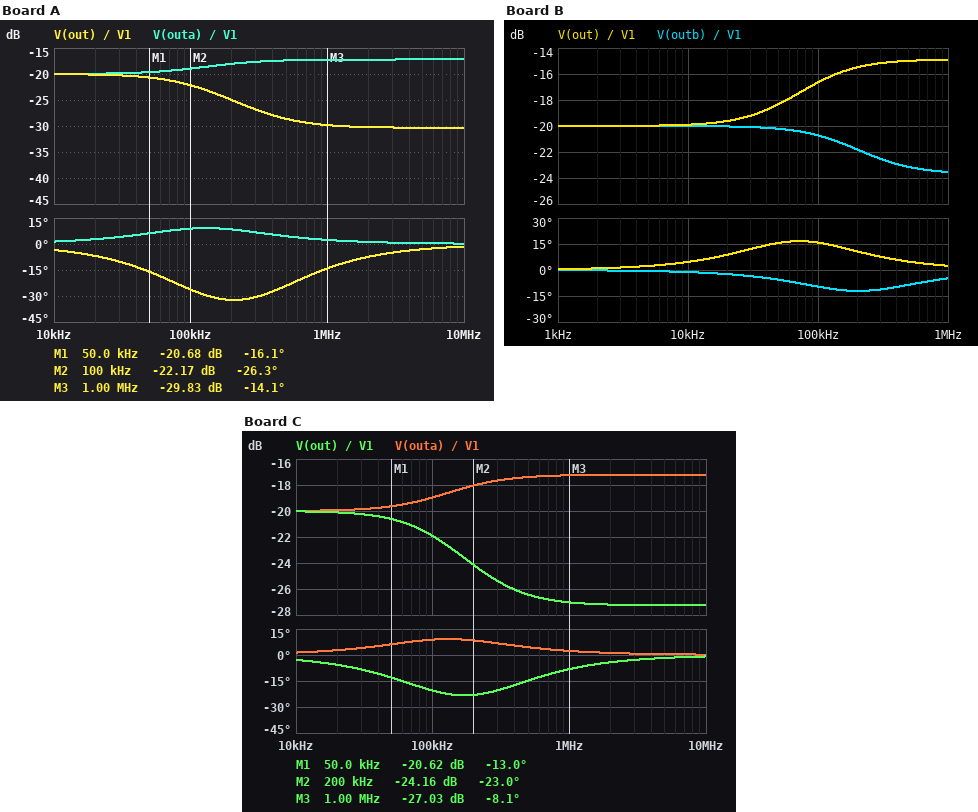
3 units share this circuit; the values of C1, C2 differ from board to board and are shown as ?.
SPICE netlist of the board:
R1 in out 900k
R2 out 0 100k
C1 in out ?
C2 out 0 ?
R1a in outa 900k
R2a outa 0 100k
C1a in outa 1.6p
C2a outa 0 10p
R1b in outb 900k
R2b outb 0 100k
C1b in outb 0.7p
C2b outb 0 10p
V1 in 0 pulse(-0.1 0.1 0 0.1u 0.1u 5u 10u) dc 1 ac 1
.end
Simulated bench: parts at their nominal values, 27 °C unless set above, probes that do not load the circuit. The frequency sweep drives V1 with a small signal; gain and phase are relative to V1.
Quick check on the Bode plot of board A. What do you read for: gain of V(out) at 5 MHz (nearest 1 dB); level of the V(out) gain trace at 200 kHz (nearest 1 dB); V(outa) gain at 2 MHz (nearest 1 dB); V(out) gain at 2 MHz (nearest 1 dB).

-30 dB
-25 dB
-17 dB
-30 dB
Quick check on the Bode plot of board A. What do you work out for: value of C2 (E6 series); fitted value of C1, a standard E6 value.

15 pF
470 fF
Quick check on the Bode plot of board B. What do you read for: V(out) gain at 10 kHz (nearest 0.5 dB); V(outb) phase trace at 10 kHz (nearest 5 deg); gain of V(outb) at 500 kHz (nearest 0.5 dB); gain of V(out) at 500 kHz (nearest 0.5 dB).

-20.0 dB
0 deg
-23.0 dB
-15.0 dB
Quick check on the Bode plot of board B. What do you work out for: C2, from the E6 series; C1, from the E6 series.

15 pF
3.3 pF
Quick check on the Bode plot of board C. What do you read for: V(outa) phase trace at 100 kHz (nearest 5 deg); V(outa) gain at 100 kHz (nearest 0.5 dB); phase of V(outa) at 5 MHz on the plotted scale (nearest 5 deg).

10 deg
-19.0 dB
0 deg
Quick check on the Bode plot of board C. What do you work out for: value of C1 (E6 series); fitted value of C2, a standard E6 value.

680 fF
15 pF
